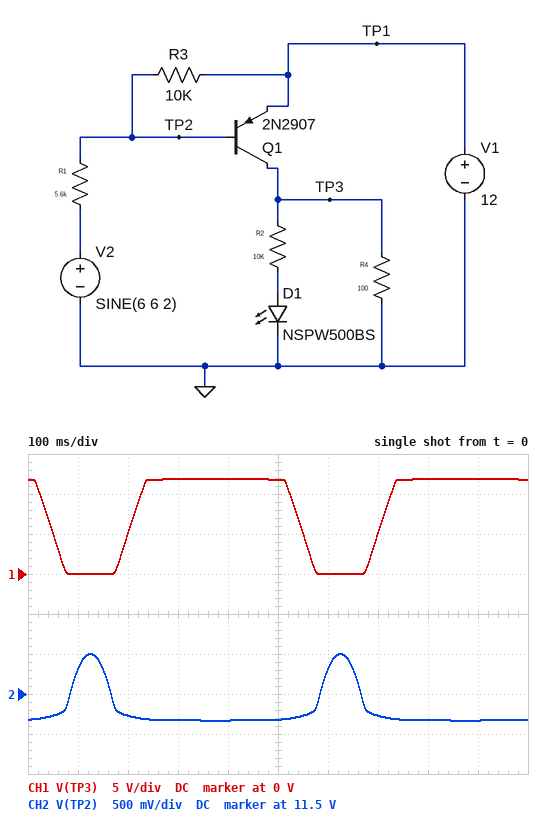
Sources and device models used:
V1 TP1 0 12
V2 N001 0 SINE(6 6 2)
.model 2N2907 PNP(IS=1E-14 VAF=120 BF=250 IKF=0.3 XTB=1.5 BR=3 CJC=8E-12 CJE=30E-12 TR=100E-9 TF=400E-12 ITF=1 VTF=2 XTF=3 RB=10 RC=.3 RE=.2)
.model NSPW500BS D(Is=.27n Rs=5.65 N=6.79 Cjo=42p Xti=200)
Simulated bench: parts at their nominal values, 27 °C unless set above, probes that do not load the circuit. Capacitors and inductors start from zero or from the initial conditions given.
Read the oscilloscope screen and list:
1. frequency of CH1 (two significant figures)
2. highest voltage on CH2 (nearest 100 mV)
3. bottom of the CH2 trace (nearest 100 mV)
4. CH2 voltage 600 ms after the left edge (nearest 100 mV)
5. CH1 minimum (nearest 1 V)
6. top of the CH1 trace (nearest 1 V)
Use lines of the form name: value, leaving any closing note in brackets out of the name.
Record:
frequency of CH1: 2.0 Hz
highest voltage on CH2: 12.0 V
bottom of the CH2 trace: 11.2 V
CH2 voltage 600 ms after the left edge: 11.8 V
CH1 minimum: 0 V
top of the CH1 trace: 12 V
